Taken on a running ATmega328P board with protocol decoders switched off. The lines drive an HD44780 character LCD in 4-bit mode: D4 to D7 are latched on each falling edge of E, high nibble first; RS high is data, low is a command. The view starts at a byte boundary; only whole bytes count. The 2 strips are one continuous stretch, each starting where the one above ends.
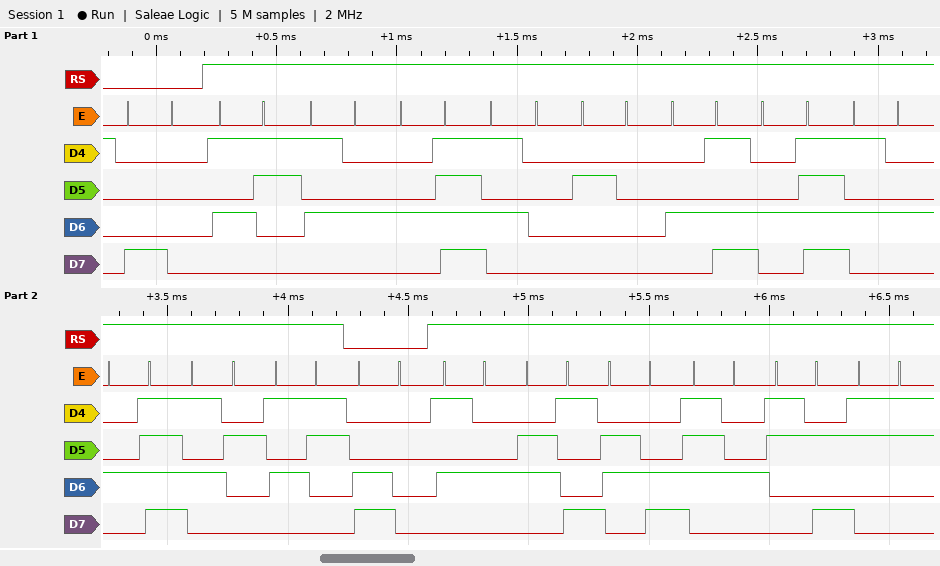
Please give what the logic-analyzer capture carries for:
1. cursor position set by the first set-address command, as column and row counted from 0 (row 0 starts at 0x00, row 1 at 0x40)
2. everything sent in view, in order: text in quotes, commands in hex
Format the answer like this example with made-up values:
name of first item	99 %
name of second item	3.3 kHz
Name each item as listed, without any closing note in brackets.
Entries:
cursor position set by the first set-address command, as column and row counted from 0	column 0, row 0
everything sent in view, in order: text in quotes, commands in hex	0x80 "STOP MOTORS" 0xC0 "Tilt:3"
